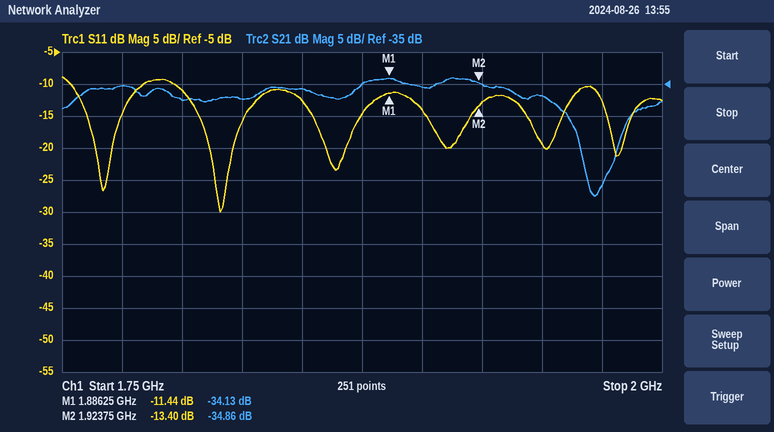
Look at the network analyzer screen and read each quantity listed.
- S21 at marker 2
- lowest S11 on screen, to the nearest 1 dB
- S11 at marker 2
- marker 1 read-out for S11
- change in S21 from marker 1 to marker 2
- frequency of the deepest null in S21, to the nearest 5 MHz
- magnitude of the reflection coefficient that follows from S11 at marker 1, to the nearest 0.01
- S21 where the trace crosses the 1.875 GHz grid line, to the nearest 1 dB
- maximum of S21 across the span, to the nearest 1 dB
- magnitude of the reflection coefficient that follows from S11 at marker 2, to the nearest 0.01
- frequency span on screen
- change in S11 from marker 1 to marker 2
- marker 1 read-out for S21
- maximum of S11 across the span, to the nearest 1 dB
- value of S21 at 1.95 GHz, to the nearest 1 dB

-34.86 dB
-30 dB
-13.40 dB
-11.44 dB
-0.73 dB
1.970 GHz
0.27
-35 dB
-34 dB
0.21
250 MHz
-1.96 dB
-34.13 dB
-9 dB
-37 dB
